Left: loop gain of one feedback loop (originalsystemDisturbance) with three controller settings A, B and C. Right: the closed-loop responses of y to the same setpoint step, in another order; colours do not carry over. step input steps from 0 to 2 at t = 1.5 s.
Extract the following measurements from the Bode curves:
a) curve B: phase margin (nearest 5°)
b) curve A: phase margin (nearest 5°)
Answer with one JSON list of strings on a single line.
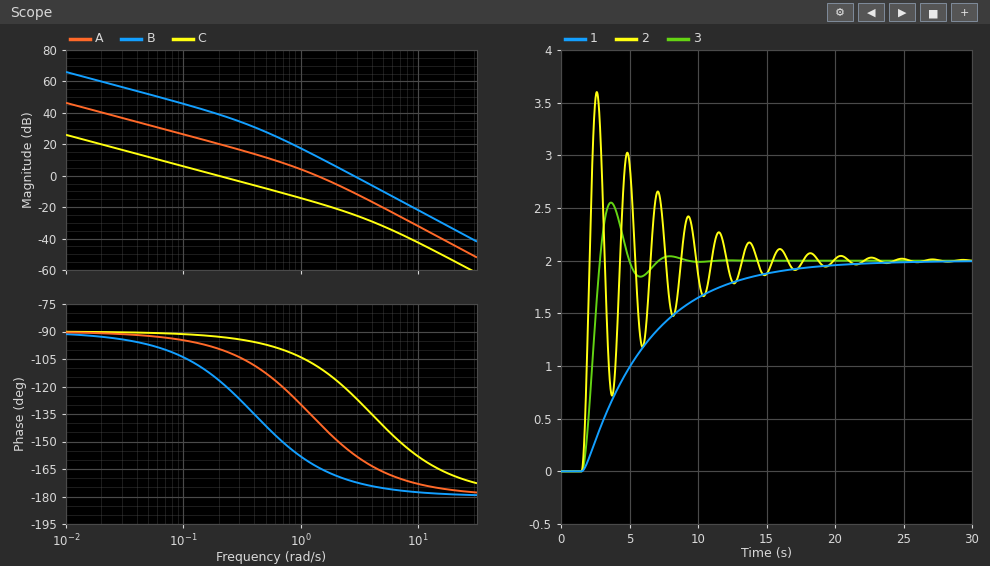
["10°", "40°"]
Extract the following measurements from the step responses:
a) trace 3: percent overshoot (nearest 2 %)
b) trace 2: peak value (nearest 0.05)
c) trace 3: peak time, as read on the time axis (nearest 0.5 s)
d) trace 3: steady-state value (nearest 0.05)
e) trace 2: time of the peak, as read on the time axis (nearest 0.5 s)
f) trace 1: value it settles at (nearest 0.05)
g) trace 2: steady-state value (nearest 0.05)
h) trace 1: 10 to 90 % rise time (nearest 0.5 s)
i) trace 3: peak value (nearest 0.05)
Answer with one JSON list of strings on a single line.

["28 %", "3.60", "3.5 s", "2.00", "2.5 s", "2.00", "2.00", "10.5 s", "2.55"]
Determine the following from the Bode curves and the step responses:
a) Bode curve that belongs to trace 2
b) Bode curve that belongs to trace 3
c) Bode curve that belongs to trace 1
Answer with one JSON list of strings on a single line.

["B", "A", "C"]
